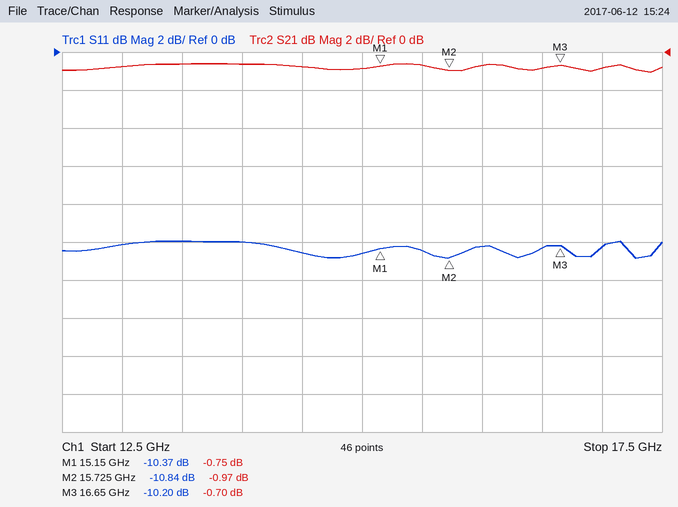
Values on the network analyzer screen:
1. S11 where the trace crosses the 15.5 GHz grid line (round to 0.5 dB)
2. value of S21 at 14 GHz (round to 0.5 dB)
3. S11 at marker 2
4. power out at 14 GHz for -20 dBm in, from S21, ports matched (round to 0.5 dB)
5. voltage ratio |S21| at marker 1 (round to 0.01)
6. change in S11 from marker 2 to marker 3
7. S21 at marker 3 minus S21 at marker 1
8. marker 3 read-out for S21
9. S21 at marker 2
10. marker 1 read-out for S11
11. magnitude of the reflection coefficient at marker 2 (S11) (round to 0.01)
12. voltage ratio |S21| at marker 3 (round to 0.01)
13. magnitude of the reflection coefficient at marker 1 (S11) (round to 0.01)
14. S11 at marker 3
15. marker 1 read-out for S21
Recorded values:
-10.5 dB
-0.5 dB
-10.84 dB
-20.5 dBm
0.92
0.64 dB
0.05 dB
-0.70 dB
-0.97 dB
-10.37 dB
0.29
0.92
0.30
-10.20 dB
-0.75 dB
